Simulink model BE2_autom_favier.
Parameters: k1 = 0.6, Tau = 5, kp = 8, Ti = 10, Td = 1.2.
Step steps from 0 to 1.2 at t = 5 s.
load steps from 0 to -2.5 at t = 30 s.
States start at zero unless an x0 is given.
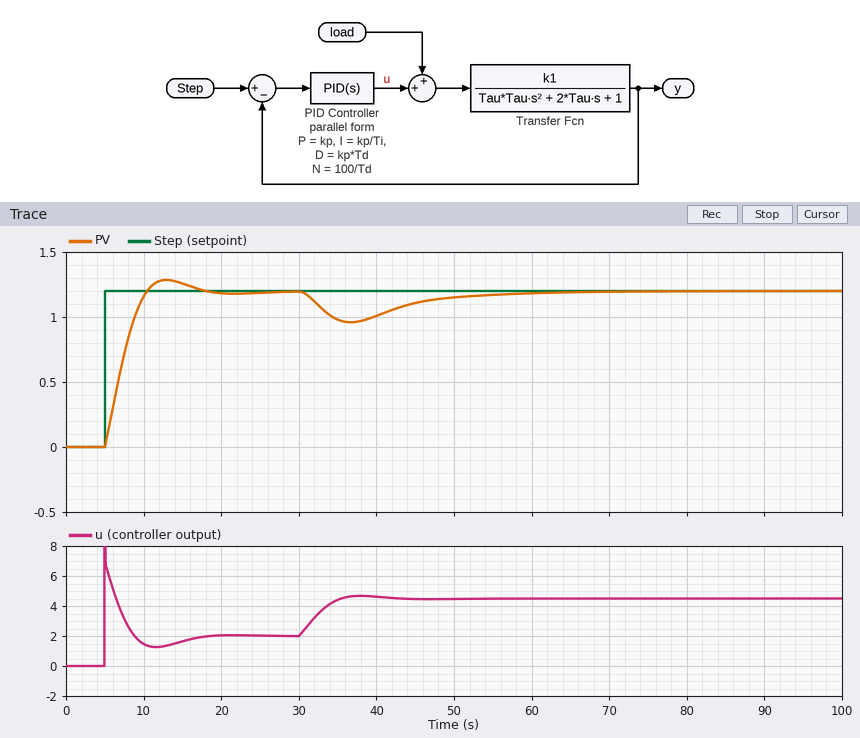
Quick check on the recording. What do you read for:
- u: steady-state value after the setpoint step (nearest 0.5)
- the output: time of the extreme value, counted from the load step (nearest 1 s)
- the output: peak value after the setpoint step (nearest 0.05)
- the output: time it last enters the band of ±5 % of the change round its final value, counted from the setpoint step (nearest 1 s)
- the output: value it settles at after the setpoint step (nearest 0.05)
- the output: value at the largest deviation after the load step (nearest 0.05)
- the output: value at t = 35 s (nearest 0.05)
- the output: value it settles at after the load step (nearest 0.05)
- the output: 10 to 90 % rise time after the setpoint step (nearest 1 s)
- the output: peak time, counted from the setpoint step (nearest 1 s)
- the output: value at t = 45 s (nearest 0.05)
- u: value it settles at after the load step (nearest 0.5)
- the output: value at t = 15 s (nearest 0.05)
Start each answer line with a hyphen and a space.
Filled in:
- 2.0
- 7 s
- 1.30
- 10 s
- 1.20
- 0.95
- 1.00
- 1.20
- 4 s
- 8 s
- 1.10
- 4.5
- 1.25
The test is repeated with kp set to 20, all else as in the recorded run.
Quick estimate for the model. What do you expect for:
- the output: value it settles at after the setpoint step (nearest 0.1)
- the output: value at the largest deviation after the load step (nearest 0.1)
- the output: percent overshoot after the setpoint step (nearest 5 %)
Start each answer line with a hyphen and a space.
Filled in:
- 1.2
- 1.1
- 10 %
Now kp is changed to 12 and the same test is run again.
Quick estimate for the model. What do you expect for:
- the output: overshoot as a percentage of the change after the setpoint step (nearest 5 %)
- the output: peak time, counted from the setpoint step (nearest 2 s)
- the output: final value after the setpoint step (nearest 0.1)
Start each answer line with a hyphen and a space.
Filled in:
- 10 %
- 6 s
- 1.2
